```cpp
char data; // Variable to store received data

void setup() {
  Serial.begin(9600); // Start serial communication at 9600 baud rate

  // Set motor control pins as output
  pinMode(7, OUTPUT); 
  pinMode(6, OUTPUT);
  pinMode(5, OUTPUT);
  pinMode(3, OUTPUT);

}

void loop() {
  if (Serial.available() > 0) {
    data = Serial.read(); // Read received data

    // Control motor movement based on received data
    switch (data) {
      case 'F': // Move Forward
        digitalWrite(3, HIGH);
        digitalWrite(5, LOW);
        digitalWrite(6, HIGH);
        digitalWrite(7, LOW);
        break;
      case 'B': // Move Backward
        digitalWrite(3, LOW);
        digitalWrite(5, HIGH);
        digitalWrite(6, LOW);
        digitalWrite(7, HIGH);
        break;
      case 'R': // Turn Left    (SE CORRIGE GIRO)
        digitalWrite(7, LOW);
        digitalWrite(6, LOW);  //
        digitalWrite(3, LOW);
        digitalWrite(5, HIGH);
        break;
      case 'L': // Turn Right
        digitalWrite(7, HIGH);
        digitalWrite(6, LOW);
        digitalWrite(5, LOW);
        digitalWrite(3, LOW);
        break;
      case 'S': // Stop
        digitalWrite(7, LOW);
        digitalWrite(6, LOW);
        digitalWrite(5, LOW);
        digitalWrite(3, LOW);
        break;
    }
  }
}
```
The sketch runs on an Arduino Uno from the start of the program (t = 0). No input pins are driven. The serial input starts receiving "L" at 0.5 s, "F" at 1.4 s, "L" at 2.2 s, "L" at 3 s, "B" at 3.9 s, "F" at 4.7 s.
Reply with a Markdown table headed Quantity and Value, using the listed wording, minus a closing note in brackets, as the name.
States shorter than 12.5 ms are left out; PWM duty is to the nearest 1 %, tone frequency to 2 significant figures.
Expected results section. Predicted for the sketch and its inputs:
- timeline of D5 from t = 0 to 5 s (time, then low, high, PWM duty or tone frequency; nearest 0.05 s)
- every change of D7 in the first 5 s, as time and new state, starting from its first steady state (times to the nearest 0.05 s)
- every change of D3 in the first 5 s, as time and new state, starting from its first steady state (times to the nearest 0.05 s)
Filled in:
| Quantity | Value |
|---|---|
| timeline of D5 from t = 0 to 5 s | 0 s low; 3.9 s high; 4.7 s low |
| every change of D7 in the first 5 s, as time and new state, starting from its first steady state | 0 s low; 0.5 s high; 1.4 s low; 2.2 s high; 4.7 s low |
| every change of D3 in the first 5 s, as time and new state, starting from its first steady state | 0 s low; 1.4 s high; 2.2 s low; 4.7 s high |
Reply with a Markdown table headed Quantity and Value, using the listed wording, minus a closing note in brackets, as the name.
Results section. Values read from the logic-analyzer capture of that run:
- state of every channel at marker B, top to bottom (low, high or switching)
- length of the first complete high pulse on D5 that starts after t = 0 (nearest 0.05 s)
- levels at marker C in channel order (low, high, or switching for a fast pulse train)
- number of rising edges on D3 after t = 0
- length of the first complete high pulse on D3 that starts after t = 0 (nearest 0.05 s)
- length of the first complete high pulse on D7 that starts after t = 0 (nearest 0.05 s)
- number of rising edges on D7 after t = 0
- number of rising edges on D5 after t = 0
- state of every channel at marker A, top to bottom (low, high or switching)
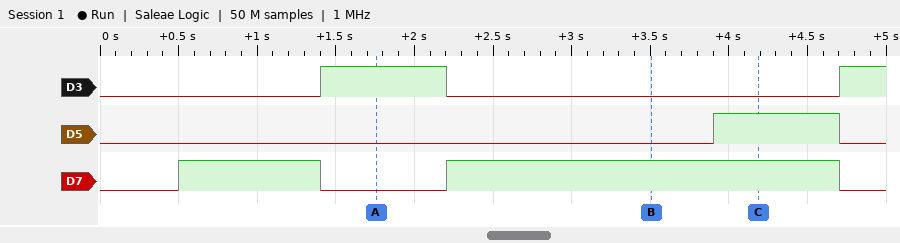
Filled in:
| Quantity | Value |
|---|---|
| state of every channel at marker B, top to bottom | D3 low, D5 low, D7 high |
| length of the first complete high pulse on D5 that starts after t = 0 | 0.80 s |
| levels at marker C in channel order | D3 low, D5 high, D7 high |
| number of rising edges on D3 after t = 0 | 2 |
| length of the first complete high pulse on D3 that starts after t = 0 | 0.80 s |
| length of the first complete high pulse on D7 that starts after t = 0 | 0.90 s |
| number of rising edges on D7 after t = 0 | 2 |
| number of rising edges on D5 after t = 0 | 1 |
| state of every channel at marker A, top to bottom | D3 high, D5 low, D7 low |
